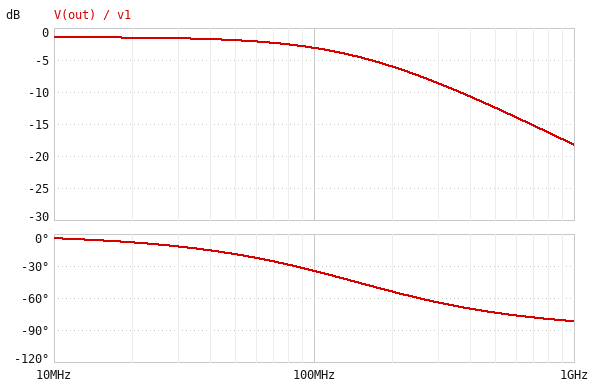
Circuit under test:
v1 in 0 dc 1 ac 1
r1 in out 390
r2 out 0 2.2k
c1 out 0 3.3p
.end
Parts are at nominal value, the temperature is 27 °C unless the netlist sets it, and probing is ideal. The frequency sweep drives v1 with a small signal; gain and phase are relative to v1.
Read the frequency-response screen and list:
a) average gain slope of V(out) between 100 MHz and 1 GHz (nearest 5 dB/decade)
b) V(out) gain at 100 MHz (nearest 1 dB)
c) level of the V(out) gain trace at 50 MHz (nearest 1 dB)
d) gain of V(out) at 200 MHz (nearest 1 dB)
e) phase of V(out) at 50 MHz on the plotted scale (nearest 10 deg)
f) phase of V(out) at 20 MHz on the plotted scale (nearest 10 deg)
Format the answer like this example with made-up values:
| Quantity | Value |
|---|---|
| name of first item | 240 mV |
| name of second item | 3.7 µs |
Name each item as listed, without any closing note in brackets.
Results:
| Quantity | Value |
|---|---|
| average gain slope of V(out) between 100 MHz and 1 GHz | -15 dB/decade |
| V(out) gain at 100 MHz | -3 dB |
| level of the V(out) gain trace at 50 MHz | -2 dB |
| gain of V(out) at 200 MHz | -6 dB |
| phase of V(out) at 50 MHz on the plotted scale | -20 deg |
| phase of V(out) at 20 MHz on the plotted scale | -10 deg |
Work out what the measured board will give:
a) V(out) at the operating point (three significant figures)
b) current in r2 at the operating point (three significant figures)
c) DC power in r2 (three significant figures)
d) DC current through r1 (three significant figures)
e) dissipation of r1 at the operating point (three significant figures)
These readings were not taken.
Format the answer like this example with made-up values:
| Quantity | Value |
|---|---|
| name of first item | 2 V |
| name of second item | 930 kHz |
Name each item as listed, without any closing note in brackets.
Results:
| Quantity | Value |
|---|---|
| V(out) at the operating point | 849 mV |
| current in r2 at the operating point | 386 µA |
| DC power in r2 | 328 µW |
| DC current through r1 | 386 µA |
| dissipation of r1 at the operating point | 58.1 µW |
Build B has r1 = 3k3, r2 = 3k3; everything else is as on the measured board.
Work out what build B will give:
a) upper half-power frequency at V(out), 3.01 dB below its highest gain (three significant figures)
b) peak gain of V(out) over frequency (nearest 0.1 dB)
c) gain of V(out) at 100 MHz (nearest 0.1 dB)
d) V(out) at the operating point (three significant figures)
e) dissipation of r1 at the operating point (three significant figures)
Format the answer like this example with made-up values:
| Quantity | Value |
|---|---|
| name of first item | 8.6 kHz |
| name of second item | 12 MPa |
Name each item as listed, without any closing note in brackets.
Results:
| Quantity | Value |
|---|---|
| upper half-power frequency at V(out), 3.01 dB below its highest gain | 29.2 MHz |
| peak gain of V(out) over frequency | -6.0 dB |
| gain of V(out) at 100 MHz | -17.1 dB |
| V(out) at the operating point | 500 mV |
| dissipation of r1 at the operating point | 75.8 µW |
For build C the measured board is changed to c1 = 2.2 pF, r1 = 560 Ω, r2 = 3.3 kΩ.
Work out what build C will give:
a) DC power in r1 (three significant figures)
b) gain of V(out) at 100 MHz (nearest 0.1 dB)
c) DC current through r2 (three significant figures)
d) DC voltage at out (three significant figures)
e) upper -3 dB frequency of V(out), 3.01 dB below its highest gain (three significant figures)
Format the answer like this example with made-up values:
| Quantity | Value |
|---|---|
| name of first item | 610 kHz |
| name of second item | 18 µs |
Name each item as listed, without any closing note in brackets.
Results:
| Quantity | Value |
|---|---|
| DC power in r1 | 37.6 µW |
| gain of V(out) at 100 MHz | -2.9 dB |
| DC current through r2 | 259 µA |
| DC voltage at out | 855 mV |
| upper -3 dB frequency of V(out), 3.01 dB below its highest gain | 151 MHz |
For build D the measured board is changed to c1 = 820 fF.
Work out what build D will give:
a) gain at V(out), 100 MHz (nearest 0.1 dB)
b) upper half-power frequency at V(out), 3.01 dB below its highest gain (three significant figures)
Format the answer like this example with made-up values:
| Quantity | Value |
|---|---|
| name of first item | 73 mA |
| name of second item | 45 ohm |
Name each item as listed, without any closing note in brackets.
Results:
| Quantity | Value |
|---|---|
| gain at V(out), 100 MHz | -1.5 dB |
| upper half-power frequency at V(out), 3.01 dB below its highest gain | 586 MHz |
